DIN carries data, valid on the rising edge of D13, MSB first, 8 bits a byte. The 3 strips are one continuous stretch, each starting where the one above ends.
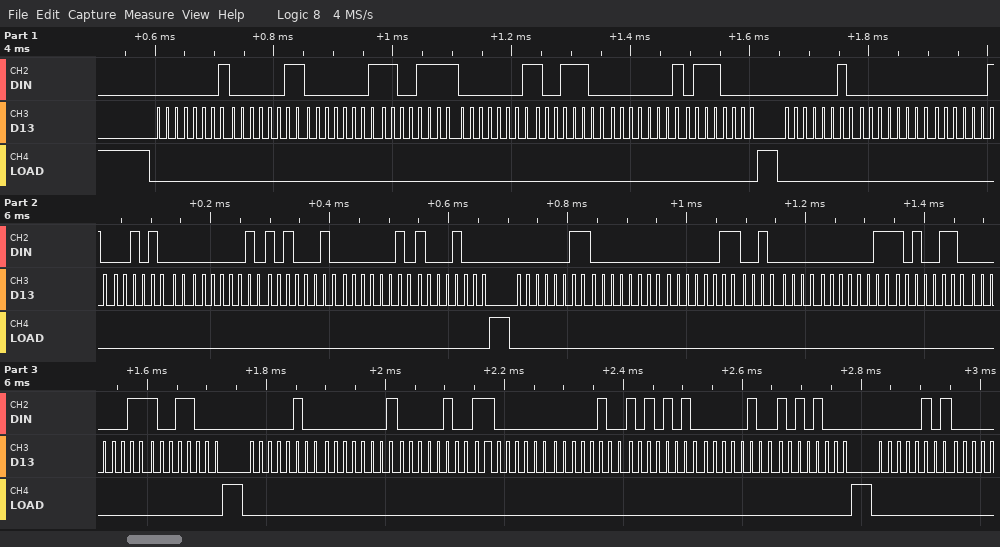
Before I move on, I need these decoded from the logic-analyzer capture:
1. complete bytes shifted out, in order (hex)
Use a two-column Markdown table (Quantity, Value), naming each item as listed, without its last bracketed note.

| Quantity | Value |
|---|---|
| complete bytes shifted out, in order | 01 03 01 CF 01 9C 01 70 02 00 02 28 02 A2 02 88 03 00 03 20 03 A6 03 98 04 01 04 C0 04 AA 04 A8 05 |
